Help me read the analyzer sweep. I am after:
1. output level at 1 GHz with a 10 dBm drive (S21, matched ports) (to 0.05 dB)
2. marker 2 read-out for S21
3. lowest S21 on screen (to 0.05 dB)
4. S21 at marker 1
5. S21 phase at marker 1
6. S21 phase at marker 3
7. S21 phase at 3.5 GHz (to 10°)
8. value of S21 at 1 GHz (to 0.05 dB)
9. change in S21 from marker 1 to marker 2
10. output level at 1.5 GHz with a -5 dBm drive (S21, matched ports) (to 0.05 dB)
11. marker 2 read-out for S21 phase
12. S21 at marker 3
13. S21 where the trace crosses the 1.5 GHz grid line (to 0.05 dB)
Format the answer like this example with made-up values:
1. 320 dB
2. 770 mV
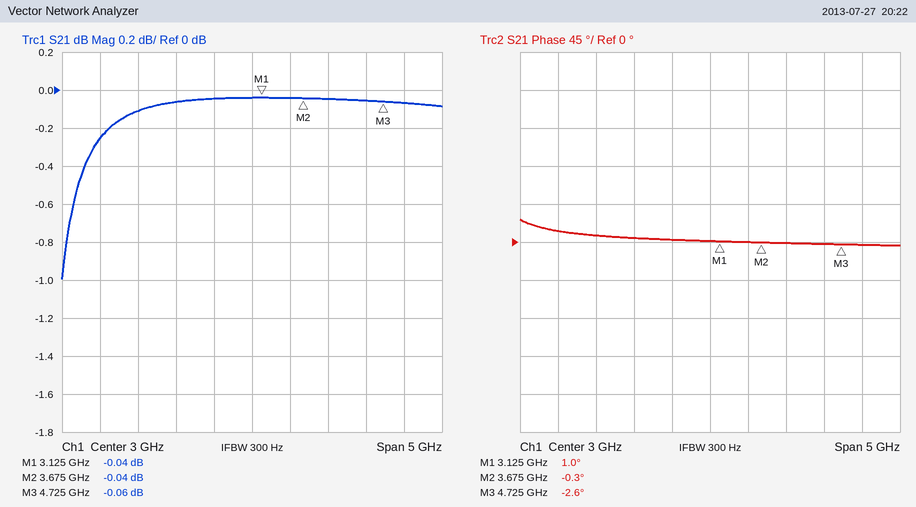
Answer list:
1. 9.75 dBm
2. -0.04 dB
3. -1.00 dB
4. -0.04 dB
5. 1.0°
6. -2.6°
7. 0°
8. -0.25 dB
9. 0.00 dB
10. -5.10 dBm
11. -0.3°
12. -0.06 dB
13. -0.10 dB
